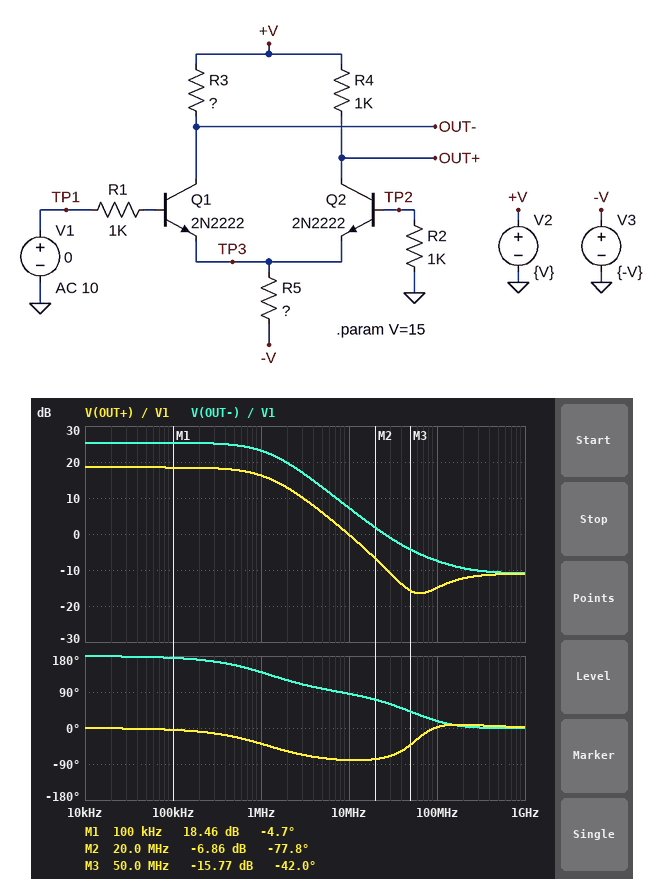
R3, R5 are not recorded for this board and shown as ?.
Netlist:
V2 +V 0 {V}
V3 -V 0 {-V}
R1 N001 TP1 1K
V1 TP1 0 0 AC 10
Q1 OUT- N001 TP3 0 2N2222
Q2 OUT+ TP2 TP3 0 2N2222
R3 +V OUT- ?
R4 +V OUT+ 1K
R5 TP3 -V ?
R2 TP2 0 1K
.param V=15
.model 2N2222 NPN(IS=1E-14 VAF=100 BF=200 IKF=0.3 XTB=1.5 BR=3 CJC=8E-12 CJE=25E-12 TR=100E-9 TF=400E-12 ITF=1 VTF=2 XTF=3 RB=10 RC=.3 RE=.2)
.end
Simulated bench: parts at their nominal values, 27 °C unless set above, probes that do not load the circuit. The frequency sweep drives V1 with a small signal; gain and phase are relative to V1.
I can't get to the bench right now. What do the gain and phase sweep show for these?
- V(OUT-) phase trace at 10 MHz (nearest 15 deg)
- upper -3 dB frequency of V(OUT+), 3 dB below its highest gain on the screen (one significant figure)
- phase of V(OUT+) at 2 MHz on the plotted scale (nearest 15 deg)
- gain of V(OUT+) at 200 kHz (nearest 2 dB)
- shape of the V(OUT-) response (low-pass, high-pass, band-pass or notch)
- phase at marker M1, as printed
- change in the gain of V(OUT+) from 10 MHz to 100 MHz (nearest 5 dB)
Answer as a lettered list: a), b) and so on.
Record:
a) 90 deg
b) 1 MHz
c) -60 deg
d) 18 dB
e) low-pass
f) -4.7 deg
g) -15 dB
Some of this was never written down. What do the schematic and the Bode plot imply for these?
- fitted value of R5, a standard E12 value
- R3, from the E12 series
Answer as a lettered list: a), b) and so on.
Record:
a) 15 kΩ
b) 2.2 kΩ
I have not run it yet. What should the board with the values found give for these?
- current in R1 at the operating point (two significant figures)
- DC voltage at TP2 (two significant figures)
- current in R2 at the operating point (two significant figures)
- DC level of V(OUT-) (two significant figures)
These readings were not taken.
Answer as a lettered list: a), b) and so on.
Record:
a) 2.1 µA
b) -2.1 mV
c) 2.1 µA
d) 14 V
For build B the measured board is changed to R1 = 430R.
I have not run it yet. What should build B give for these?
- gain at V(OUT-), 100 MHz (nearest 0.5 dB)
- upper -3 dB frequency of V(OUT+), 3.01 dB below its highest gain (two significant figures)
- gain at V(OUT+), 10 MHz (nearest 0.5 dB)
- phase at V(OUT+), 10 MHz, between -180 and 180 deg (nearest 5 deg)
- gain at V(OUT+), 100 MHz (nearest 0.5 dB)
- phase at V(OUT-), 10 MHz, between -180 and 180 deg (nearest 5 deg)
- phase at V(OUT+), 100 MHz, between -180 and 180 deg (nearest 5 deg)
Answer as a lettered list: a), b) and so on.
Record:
a) -3.0 dB
b) 1.8 MHz
c) 3.5 dB
d) -75 deg
e) -10.5 dB
f) 90 deg
g) 5 deg
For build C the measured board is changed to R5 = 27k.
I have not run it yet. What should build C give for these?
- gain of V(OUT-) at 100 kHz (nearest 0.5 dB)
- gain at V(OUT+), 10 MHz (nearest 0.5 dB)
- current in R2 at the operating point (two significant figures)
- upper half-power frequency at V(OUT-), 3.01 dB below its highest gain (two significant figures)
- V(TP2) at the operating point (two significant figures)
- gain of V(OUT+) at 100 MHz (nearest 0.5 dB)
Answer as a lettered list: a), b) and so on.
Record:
a) 20.5 dB
b) -2.5 dB
c) 1.2 µA
d) 1.7 MHz
e) -1.2 mV
f) -14.0 dB
